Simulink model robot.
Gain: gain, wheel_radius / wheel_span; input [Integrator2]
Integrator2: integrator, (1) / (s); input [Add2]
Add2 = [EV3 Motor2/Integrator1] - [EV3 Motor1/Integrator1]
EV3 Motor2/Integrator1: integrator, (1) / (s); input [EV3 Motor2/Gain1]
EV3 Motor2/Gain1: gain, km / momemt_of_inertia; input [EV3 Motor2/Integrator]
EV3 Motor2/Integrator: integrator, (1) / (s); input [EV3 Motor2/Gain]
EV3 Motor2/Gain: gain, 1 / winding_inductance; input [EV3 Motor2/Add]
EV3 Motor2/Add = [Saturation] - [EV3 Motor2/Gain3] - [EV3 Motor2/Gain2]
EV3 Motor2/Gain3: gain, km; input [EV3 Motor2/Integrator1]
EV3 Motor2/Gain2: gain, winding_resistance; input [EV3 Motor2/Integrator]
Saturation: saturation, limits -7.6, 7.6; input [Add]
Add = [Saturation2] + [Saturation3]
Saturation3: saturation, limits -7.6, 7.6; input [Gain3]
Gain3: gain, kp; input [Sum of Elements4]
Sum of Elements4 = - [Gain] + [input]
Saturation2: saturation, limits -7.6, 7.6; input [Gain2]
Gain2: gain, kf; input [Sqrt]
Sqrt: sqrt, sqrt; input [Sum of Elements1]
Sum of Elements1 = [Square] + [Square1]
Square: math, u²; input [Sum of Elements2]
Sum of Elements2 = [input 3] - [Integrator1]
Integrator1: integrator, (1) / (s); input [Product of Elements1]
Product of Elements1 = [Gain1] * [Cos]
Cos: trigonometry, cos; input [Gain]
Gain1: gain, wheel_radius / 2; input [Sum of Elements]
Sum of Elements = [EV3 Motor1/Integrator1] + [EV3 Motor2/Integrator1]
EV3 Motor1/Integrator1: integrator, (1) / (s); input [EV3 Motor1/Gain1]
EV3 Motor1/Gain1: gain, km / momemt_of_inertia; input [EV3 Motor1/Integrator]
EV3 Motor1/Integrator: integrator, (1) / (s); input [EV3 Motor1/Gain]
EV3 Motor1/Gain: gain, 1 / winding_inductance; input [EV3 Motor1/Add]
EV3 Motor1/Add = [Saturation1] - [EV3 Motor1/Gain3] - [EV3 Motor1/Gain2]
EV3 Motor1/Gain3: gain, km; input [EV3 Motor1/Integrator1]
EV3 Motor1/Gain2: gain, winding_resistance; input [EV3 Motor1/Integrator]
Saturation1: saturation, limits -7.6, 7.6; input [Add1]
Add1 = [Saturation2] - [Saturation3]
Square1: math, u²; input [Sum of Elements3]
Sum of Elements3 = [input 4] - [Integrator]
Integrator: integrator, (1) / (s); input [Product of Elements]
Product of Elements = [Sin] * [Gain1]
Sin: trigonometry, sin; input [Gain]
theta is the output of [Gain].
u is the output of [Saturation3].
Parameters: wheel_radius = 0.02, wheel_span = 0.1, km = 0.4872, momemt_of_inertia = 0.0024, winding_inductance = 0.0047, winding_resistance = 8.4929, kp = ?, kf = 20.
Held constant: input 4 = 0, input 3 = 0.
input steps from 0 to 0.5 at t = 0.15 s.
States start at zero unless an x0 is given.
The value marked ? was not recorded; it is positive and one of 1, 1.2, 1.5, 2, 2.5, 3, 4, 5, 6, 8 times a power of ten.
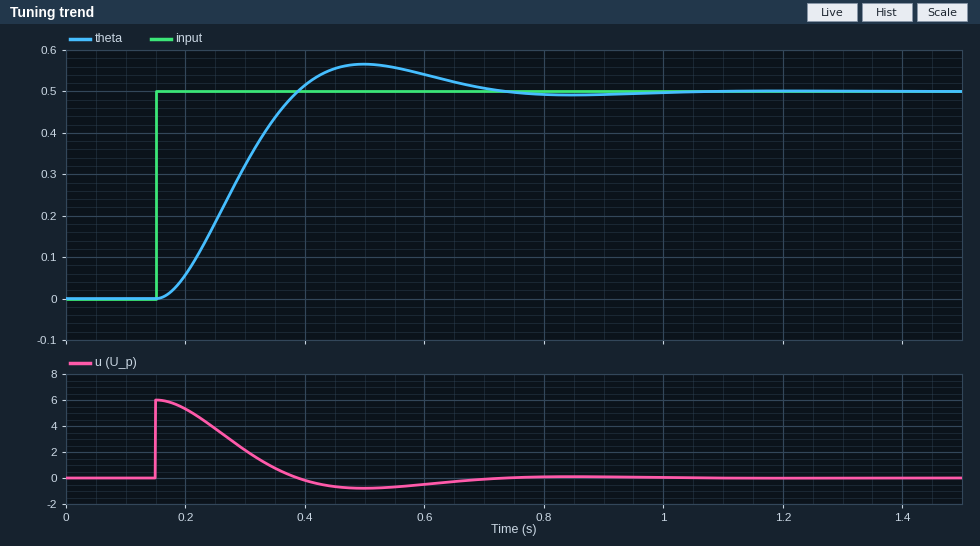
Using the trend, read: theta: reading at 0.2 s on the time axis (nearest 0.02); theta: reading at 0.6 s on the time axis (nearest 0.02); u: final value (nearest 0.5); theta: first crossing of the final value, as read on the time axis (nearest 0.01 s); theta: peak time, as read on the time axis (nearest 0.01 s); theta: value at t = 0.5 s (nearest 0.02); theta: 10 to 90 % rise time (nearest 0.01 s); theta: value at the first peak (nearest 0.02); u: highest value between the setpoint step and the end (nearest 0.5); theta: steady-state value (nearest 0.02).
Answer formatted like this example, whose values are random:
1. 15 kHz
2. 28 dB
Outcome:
1. 0.06
2. 0.54
3. 0.0
4. 0.39 s
5. 0.50 s
6. 0.56
7. 0.16 s
8. 0.56
9. 6.0
10. 0.50
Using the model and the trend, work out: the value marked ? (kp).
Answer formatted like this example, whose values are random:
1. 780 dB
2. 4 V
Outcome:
1. 12
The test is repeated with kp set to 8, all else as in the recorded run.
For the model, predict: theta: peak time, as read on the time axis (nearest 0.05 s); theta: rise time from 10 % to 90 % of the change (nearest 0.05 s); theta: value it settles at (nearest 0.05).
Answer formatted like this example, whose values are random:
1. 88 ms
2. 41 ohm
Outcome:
1. 0.65 s
2. 0.25 s
3. 0.50
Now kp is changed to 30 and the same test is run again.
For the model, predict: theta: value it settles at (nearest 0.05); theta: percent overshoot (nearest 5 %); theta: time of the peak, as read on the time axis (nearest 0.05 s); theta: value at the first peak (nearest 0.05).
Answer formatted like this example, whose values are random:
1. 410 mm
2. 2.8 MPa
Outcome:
1. 0.50
2. 25 %
3. 0.40 s
4. 0.65
